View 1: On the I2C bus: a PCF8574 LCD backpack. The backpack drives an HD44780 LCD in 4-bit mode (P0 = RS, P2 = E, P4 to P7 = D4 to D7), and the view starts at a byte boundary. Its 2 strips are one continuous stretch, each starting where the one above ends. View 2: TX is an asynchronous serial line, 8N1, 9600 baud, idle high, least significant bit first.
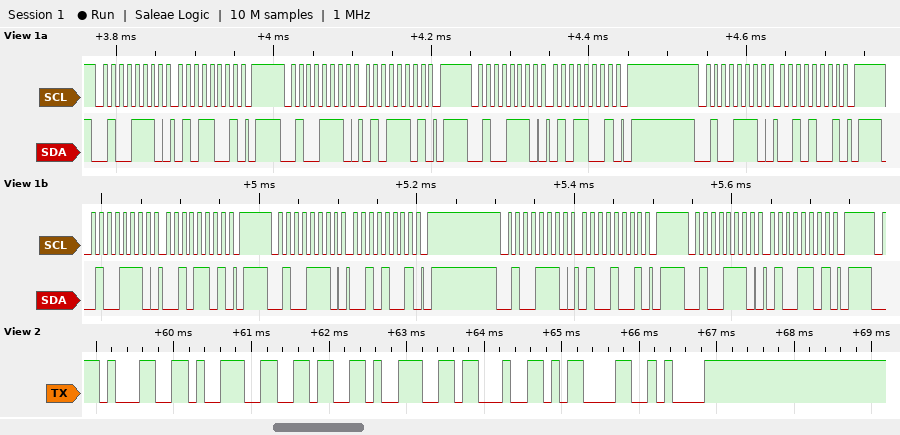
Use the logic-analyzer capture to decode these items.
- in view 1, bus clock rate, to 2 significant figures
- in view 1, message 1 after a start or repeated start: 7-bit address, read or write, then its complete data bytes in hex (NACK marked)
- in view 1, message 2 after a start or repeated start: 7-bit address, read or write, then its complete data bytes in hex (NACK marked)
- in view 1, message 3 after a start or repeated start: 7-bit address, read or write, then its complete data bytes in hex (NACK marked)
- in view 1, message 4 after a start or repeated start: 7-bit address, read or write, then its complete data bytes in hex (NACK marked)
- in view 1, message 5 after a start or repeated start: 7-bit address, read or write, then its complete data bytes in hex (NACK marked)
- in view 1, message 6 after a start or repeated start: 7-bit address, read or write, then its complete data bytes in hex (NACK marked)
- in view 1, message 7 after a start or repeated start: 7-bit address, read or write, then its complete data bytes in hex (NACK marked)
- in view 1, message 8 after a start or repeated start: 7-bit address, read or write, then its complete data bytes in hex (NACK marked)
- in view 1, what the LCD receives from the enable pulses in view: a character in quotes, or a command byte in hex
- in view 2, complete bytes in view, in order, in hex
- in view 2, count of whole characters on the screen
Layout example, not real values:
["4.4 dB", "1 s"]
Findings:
["100 kHz", "0x27 write: 59", "0x27 write: 5D", "0x27 write: 59", "0x27 write: 29", "0x27 write: 2D", "0x27 write: 29", "0x27 write: 49", "0x27 write: 4D", "'R'", "31 39 36 39 23 0D 0A", "7"]
